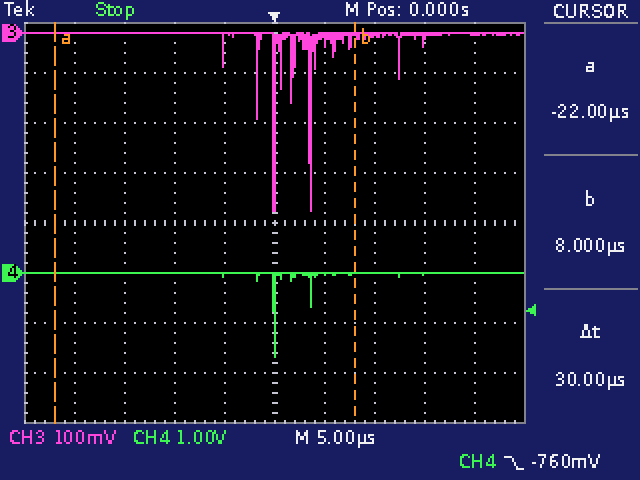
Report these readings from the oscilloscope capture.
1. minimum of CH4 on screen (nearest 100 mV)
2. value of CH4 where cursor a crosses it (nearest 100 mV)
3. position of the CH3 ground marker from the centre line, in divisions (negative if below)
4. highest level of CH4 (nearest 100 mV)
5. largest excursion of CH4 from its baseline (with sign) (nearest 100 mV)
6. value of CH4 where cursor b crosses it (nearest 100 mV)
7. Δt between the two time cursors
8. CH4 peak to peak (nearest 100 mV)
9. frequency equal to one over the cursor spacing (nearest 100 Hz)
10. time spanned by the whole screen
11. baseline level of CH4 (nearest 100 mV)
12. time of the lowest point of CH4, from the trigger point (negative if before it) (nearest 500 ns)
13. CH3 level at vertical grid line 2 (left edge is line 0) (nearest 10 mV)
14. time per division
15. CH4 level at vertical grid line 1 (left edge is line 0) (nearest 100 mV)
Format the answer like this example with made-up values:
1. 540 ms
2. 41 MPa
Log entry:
1. -1.7 V
2. 0.0 V
3. +3.8 div
4. 0.0 V
5. -1.7 V
6. 0.0 V
7. 30 µs
8. 1.7 V
9. 33.3 kHz
10. 50 µs
11. 0.0 V
12. 0.0 µs
13. 0 mV
14. 5 µs
15. 0.0 V
